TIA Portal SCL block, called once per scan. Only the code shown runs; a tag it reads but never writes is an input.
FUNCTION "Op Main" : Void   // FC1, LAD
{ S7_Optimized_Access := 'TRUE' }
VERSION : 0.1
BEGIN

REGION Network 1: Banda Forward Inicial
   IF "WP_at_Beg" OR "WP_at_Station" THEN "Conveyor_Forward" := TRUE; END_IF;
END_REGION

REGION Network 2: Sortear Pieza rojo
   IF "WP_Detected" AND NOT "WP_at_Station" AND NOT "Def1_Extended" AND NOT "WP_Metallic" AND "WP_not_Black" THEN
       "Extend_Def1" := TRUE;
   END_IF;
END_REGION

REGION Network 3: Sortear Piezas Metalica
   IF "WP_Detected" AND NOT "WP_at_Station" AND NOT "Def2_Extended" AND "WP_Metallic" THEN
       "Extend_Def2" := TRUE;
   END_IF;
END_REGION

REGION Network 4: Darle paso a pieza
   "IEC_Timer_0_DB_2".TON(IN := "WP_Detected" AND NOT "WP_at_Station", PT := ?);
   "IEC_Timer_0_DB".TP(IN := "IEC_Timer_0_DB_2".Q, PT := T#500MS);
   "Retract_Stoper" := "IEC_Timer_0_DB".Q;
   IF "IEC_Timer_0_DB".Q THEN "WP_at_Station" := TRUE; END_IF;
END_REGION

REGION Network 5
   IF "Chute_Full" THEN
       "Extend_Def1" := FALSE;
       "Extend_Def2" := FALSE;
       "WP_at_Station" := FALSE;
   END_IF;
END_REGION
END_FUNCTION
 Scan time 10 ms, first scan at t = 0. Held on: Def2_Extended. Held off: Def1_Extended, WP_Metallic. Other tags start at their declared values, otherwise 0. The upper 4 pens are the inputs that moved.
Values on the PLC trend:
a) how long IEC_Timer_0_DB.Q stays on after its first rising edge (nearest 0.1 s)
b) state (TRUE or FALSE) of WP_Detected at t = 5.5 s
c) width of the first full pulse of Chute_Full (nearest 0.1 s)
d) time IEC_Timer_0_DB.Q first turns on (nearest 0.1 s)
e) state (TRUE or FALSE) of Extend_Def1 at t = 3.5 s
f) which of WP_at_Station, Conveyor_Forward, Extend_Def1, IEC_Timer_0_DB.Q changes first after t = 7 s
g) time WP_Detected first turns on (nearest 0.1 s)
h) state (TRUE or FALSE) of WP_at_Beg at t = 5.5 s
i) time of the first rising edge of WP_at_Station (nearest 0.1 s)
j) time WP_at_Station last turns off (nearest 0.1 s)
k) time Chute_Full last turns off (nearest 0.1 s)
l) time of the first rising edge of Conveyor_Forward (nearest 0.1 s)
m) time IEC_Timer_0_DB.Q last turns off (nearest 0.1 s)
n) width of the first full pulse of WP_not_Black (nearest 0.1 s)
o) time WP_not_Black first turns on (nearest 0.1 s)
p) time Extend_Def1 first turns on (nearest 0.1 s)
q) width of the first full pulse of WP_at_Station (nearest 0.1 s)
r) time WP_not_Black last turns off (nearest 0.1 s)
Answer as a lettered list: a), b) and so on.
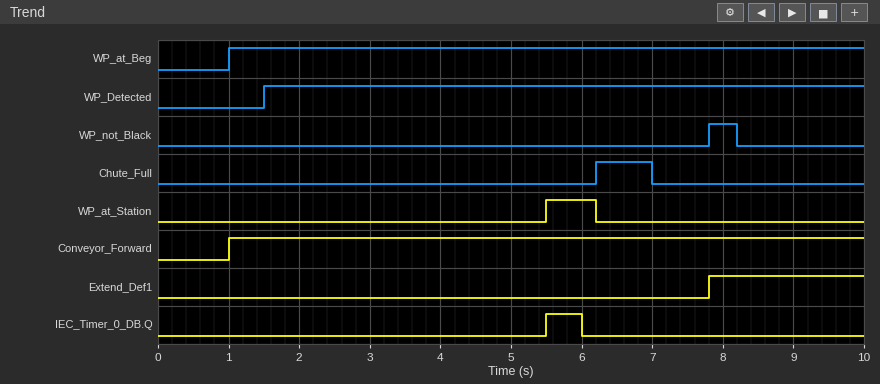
a) 0.5 s
b) TRUE
c) 0.8 s
d) 5.5 s
e) FALSE
f) Extend_Def1
g) 1.5 s
h) TRUE
i) 5.5 s
j) 6.2 s
k) 7.0 s
l) 1.0 s
m) 6.0 s
n) 0.4 s
o) 7.8 s
p) 7.8 s
q) 0.7 s
r) 8.2 s
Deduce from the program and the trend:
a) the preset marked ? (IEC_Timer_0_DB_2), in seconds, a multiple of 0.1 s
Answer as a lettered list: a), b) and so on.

a) 4.0 s
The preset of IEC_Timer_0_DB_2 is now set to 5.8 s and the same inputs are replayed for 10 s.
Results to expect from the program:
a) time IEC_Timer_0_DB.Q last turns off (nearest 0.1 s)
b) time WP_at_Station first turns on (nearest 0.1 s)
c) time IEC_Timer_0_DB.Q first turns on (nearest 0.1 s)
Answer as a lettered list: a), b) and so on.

a) 7.8 s
b) 7.3 s
c) 7.3 s
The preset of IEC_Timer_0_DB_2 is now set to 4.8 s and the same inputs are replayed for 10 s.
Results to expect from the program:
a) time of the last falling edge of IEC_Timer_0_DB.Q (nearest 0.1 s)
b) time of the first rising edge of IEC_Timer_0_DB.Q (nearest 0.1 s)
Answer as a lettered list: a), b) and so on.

a) 6.8 s
b) 6.3 s
